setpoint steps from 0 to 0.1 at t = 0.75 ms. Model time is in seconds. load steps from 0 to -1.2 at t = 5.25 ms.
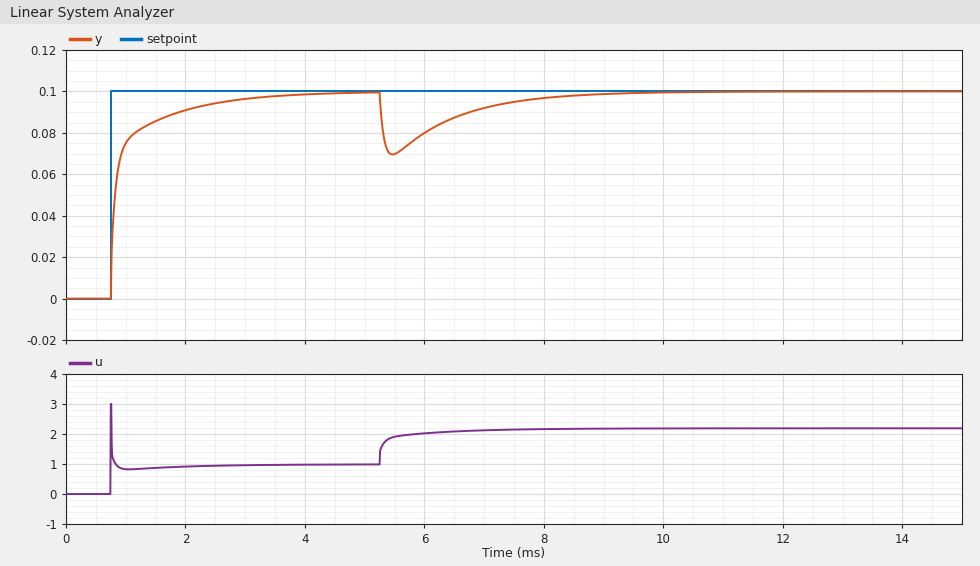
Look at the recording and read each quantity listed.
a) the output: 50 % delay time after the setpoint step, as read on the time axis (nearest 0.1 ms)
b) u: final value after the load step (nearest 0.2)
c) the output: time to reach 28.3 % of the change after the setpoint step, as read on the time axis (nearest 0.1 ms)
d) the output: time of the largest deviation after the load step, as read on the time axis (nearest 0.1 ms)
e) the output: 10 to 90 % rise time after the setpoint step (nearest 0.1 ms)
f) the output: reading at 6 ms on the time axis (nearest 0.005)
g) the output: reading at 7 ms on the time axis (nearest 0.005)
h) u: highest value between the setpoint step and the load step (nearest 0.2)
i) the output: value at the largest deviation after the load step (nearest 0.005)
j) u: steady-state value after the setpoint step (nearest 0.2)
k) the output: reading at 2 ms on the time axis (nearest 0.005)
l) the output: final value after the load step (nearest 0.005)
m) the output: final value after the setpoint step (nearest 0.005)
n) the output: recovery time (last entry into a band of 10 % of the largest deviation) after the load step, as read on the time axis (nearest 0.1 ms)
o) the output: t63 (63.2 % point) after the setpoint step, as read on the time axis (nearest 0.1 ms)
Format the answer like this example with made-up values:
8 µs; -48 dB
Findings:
0.8 ms; 2.2; 0.8 ms; 5.5 ms; 1.1 ms; 0.080; 0.090; 3.0; 0.070; 1.0; 0.090; 0.100; 0.100; 8.1 ms; 0.9 ms
